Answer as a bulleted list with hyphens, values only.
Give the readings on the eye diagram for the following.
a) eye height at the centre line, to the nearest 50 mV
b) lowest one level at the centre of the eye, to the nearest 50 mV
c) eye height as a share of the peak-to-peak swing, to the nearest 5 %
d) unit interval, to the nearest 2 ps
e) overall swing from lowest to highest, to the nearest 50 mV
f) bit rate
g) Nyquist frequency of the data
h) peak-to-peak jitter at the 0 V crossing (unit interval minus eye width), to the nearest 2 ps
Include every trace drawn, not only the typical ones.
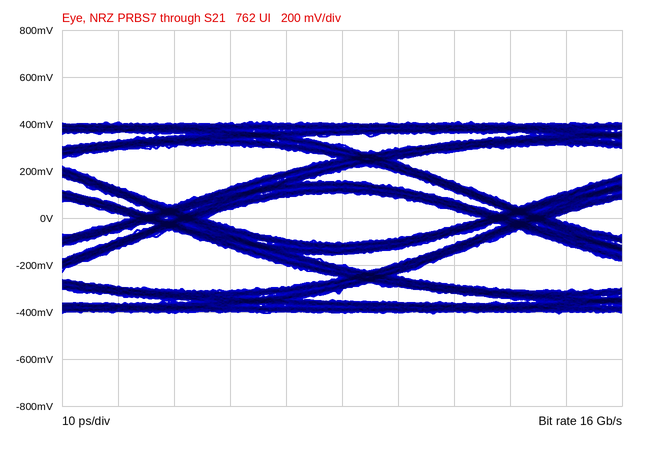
- 200 mV
- 100 mV
- 25 %
- 62 ps
- 800 mV
- 16 Gb/s
- 8 GHz
- 14 ps
